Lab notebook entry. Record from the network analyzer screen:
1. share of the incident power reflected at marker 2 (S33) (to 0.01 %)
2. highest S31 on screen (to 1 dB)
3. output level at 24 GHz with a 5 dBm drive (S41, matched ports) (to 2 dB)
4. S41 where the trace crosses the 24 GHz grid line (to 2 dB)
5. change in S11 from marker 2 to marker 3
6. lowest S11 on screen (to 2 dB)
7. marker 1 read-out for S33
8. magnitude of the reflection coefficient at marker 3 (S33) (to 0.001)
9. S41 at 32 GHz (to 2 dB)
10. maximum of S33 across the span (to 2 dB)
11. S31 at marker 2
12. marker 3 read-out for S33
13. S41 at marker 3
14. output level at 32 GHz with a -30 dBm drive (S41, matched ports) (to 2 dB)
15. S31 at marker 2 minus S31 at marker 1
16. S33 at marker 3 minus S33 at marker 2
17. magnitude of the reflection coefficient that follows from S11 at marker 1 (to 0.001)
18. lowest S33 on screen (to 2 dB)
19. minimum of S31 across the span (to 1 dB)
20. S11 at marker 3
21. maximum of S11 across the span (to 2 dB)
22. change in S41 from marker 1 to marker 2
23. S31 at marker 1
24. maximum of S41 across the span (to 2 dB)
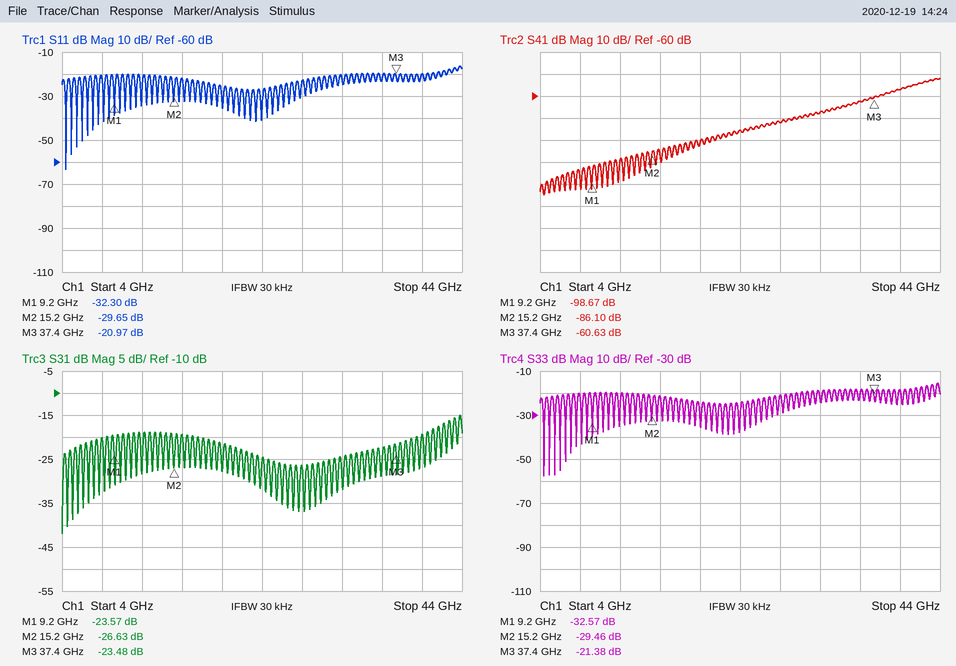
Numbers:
0.11 %
-15 dB
-70 dBm
-76 dB
8.68 dB
-64 dB
-32.57 dB
0.085
-68 dB
-16 dB
-26.63 dB
-21.38 dB
-60.63 dB
-98 dBm
-3.06 dB
8.08 dB
0.024
-58 dB
-42 dB
-20.97 dB
-16 dB
12.57 dB
-23.57 dB
-52 dB
